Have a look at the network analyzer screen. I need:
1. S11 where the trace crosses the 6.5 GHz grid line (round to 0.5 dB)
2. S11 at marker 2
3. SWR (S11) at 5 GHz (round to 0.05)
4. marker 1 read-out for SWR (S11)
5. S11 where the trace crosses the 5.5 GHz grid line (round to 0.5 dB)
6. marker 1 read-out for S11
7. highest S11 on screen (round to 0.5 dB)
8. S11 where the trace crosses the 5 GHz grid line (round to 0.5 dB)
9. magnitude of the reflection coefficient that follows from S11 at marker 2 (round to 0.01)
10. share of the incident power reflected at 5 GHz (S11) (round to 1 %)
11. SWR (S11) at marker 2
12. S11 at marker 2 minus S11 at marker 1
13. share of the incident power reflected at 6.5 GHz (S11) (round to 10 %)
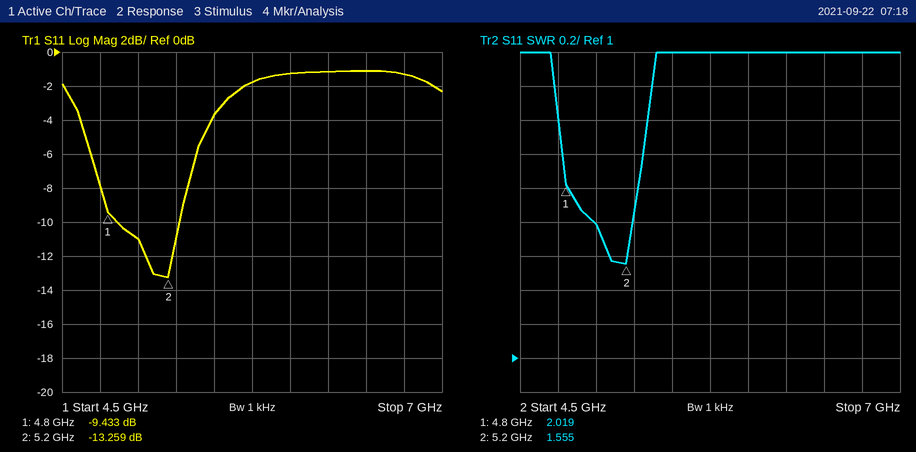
-1.0 dB
-13.259 dB
1.80
2.019
-3.5 dB
-9.433 dB
-1.0 dB
-11.0 dB
0.22
8 %
1.555
-3.826 dB
80 %
